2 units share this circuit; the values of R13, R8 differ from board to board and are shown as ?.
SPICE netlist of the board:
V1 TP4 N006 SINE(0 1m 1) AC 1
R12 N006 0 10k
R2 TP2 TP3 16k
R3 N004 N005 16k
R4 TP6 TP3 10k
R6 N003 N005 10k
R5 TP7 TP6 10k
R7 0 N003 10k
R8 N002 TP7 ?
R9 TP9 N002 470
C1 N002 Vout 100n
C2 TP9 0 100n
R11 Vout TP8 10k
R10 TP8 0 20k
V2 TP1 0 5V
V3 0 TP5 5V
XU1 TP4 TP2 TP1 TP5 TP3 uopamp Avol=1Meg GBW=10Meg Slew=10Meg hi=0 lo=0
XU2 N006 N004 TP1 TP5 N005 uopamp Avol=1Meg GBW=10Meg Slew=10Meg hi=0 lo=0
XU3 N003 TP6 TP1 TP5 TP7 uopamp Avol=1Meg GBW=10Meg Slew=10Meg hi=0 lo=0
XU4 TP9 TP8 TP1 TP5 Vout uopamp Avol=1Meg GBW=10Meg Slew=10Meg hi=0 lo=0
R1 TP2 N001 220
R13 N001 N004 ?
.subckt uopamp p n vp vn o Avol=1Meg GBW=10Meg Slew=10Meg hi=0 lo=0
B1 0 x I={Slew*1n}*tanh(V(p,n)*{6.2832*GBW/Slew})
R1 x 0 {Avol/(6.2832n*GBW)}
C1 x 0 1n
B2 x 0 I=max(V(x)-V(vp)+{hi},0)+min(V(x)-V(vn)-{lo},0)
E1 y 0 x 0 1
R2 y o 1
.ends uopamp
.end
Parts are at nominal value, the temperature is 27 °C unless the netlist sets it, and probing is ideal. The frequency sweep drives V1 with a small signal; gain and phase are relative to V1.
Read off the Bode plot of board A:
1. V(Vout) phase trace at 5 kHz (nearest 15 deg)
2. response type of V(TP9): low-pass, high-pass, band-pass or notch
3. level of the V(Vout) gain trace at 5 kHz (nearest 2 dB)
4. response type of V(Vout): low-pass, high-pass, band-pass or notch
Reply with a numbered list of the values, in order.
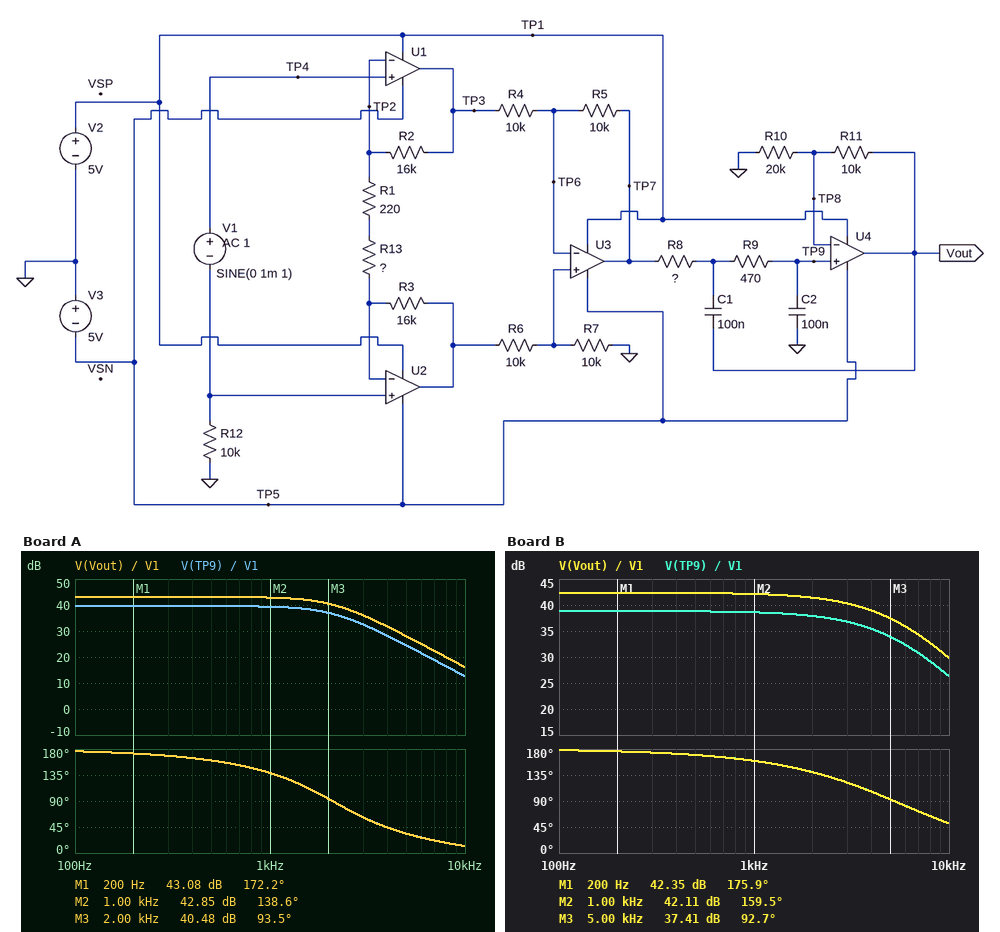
1. 30 deg
2. low-pass
3. 28 dB
4. low-pass
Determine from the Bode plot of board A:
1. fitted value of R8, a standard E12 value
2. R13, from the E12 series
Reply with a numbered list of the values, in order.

1. 1.2 kΩ
2. 120 Ω
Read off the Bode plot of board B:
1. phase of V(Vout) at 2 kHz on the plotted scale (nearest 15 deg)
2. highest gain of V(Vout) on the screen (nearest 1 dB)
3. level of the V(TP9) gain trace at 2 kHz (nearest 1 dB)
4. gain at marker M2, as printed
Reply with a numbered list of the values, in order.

1. 135 deg
2. 42 dB
3. 38 dB
4. 42.11 dB
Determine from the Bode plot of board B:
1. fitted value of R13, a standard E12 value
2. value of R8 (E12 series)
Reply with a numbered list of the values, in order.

1. 150 Ω
2. 180 Ω
